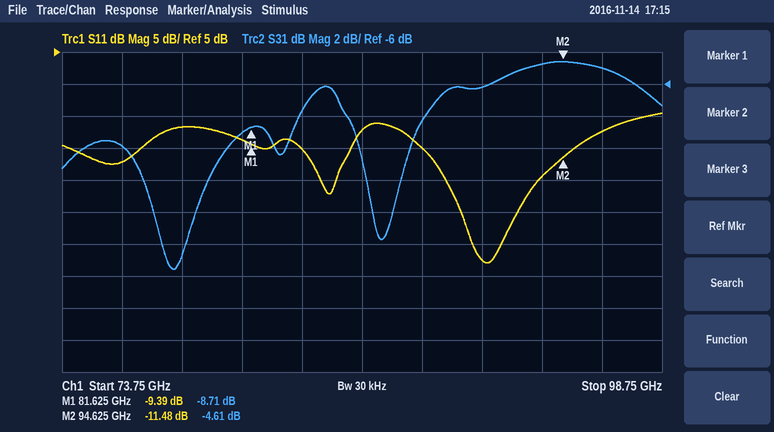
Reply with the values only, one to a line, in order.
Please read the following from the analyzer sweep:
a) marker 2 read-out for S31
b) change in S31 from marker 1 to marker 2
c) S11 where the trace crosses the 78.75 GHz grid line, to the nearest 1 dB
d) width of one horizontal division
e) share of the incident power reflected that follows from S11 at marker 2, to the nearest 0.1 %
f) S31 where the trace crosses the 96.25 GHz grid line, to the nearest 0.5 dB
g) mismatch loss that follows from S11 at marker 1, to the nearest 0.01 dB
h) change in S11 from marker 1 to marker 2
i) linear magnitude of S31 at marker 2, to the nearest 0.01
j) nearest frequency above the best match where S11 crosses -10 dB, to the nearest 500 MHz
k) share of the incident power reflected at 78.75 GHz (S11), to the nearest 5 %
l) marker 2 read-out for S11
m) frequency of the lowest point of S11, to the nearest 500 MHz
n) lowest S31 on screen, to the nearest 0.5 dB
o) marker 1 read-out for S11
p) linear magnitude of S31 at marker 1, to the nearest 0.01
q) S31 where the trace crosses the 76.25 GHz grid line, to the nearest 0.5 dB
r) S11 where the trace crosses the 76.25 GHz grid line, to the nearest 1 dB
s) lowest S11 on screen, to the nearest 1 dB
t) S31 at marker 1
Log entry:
-4.61 dB
4.10 dB
-7 dB
2.5 GHz
7.1 %
-5.0 dB
0.53 dB
-2.09 dB
0.59
95.0 GHz
20 %
-11.48 dB
91.5 GHz
-17.5 dB
-9.39 dB
0.37
-10.0 dB
-12 dB
-28 dB
-8.71 dB
